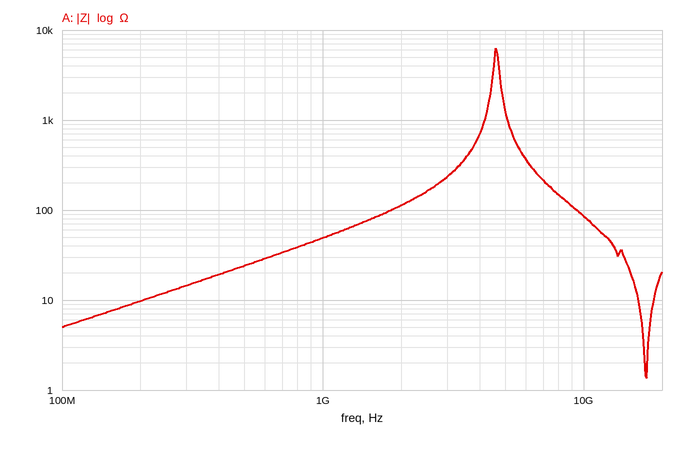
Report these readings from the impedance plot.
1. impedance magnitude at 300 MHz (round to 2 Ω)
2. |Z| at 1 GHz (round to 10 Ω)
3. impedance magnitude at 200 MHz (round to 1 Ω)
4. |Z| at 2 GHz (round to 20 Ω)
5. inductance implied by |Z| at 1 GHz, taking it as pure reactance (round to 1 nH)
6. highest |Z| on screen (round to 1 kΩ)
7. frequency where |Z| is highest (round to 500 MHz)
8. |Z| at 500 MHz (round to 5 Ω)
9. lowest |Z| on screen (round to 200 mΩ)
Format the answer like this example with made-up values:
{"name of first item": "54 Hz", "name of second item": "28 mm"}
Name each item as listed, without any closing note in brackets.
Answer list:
{"impedance magnitude at 300 MHz": "14 Ω", "|Z| at 1 GHz": "50 Ω", "impedance magnitude at 200 MHz": "10 Ω", "|Z| at 2 GHz": "120 Ω", "inductance implied by |Z| at 1 GHz, taking it as pure reactance": "8 nH", "highest |Z| on screen": "6 kΩ", "frequency where |Z| is highest": "4.5 GHz", "|Z| at 500 MHz": "25 Ω", "lowest |Z| on screen": "1.4 Ω"}
